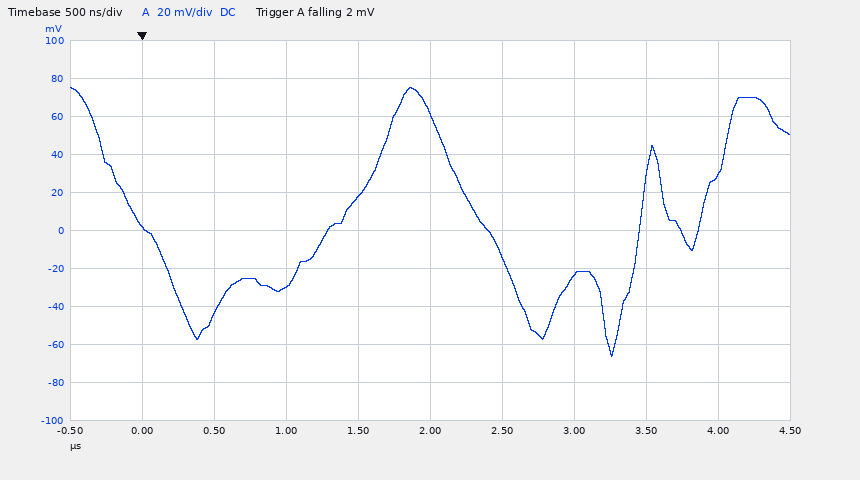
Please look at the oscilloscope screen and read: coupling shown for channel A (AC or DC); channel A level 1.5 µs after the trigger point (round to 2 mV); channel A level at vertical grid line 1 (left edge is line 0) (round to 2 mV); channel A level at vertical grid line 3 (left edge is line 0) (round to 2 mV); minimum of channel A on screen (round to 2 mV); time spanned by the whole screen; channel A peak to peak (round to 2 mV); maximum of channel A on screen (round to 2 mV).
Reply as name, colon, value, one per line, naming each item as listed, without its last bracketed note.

coupling shown for channel A: DC
channel A level 1.5 µs after the trigger point: 18 mV
channel A level at vertical grid line 1 (left edge is line 0): 2 mV
channel A level at vertical grid line 3 (left edge is line 0): -30 mV
minimum of channel A on screen: -66 mV
time spanned by the whole screen: 5 µs
channel A peak to peak: 142 mV
maximum of channel A on screen: 76 mV
